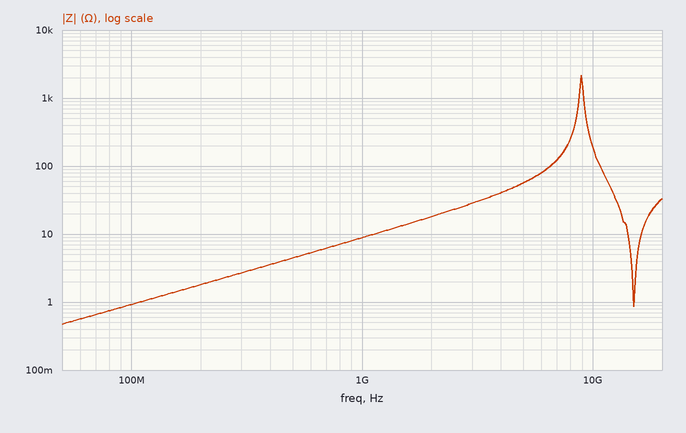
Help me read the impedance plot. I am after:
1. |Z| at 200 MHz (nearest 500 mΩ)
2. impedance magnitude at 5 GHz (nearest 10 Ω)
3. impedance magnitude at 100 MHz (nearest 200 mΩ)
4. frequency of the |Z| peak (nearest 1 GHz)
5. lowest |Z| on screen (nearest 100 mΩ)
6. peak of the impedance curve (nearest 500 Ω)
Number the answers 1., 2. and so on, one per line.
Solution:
1. 2.0 Ω
2. 60 Ω
3. 1.0 Ω
4. 9 GHz
5. 500 mΩ
6. 2.0 kΩ
